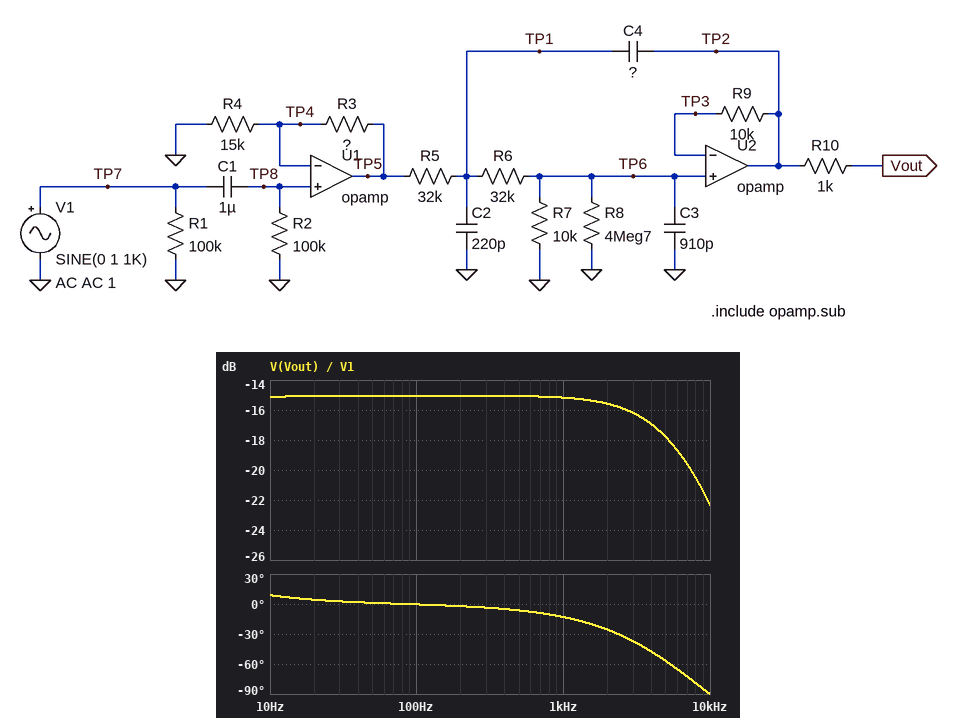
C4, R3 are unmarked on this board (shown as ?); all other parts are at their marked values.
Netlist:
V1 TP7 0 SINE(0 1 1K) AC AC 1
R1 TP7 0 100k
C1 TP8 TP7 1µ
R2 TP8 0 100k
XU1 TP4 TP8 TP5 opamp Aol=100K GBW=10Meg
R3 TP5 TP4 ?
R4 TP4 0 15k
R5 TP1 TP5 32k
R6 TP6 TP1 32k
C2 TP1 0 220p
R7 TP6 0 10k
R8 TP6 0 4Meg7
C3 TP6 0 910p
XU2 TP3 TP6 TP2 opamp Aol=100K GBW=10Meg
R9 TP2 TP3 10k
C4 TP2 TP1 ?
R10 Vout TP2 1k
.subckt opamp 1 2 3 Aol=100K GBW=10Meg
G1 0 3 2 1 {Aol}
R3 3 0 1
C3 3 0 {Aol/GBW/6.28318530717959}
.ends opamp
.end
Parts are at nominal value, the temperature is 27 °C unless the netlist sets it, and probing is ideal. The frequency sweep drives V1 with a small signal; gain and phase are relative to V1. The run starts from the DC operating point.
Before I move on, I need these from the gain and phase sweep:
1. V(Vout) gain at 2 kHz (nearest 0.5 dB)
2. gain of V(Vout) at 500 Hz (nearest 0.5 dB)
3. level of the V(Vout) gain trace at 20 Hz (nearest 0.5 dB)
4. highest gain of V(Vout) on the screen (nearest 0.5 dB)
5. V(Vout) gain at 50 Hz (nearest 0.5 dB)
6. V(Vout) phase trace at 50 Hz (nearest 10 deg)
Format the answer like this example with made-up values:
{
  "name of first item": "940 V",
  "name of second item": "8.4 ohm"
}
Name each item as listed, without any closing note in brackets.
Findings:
{
  "V(Vout) gain at 2 kHz": "-15.5 dB",
  "gain of V(Vout) at 500 Hz": "-15.0 dB",
  "level of the V(Vout) gain trace at 20 Hz": "-15.0 dB",
  "highest gain of V(Vout) on the screen": "-15.0 dB",
  "V(Vout) gain at 50 Hz": "-15.0 dB",
  "V(Vout) phase trace at 50 Hz": "0 deg"
}
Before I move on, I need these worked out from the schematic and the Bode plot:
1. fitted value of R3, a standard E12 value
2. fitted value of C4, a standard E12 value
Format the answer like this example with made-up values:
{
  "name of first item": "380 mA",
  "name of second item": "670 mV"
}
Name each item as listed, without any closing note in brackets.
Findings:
{
  "fitted value of R3, a standard E12 value": "4.7 kΩ",
  "fitted value of C4, a standard E12 value": "1.8 nF"
}
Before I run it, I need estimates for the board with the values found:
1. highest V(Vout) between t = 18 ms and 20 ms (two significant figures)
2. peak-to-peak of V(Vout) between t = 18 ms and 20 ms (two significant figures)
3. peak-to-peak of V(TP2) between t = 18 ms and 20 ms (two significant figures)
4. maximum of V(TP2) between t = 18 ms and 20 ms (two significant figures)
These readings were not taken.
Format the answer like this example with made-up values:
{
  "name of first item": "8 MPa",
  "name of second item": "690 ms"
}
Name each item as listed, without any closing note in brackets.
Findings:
{
  "highest V(Vout) between t = 18 ms and 20 ms": "170 mV",
  "peak-to-peak of V(Vout) between t = 18 ms and 20 ms": "350 mV",
  "peak-to-peak of V(TP2) between t = 18 ms and 20 ms": "350 mV",
  "maximum of V(TP2) between t = 18 ms and 20 ms": "170 mV"
}
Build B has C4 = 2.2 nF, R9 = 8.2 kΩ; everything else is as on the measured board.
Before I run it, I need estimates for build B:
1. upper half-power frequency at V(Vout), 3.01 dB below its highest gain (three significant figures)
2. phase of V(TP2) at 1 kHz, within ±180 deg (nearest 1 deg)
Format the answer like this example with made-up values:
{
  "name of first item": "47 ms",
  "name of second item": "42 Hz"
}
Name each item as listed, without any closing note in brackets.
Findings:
{
  "upper half-power frequency at V(Vout), 3.01 dB below its highest gain": "4.50 kHz",
  "phase of V(TP2) at 1 kHz, within ±180 deg": "-15 deg"
}
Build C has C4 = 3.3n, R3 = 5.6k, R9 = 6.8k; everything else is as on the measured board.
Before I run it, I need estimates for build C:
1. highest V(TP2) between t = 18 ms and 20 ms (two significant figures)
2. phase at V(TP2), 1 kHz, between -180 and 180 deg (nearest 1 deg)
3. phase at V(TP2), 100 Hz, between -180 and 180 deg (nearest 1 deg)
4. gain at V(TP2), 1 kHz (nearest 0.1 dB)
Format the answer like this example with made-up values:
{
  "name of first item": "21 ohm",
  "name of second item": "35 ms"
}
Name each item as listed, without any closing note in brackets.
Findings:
{
  "highest V(TP2) between t = 18 ms and 20 ms": "180 mV",
  "phase at V(TP2), 1 kHz, between -180 and 180 deg": "-20 deg",
  "phase at V(TP2), 100 Hz, between -180 and 180 deg": "-1 deg",
  "gain at V(TP2), 1 kHz": "-15.0 dB"
}
